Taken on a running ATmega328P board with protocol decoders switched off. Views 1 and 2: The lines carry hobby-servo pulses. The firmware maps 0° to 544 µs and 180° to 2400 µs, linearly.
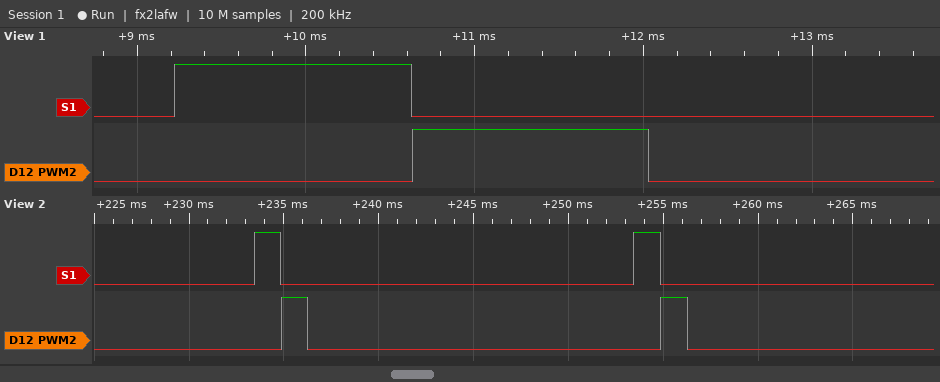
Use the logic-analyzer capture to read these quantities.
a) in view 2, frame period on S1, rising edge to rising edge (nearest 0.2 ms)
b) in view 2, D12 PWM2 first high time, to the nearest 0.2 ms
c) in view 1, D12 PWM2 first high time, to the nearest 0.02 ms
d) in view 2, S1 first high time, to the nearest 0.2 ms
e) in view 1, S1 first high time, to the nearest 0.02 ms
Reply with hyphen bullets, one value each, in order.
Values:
- 20.0 ms
- 1.4 ms
- 1.40 ms
- 1.4 ms
- 1.40 ms
